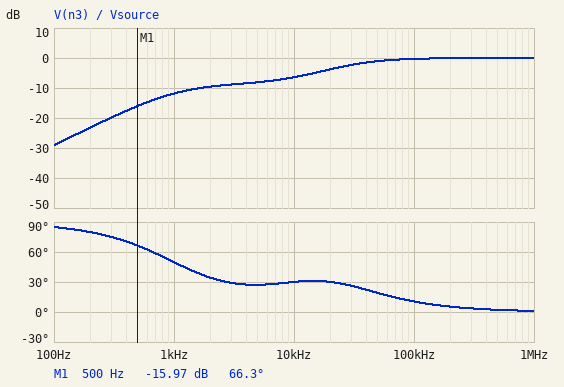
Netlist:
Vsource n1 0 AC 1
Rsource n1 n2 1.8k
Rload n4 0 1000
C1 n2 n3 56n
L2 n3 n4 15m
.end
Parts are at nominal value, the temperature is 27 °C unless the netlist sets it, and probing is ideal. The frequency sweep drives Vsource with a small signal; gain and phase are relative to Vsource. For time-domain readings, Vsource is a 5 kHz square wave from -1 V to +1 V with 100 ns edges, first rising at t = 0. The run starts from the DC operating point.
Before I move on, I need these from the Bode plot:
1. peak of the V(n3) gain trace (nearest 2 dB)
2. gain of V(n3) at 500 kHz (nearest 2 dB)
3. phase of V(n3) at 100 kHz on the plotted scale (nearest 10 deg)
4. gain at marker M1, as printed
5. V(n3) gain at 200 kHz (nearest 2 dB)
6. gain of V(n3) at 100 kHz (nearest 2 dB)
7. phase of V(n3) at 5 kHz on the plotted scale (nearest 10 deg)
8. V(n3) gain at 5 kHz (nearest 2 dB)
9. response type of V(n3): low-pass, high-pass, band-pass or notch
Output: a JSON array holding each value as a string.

["0 dB", "0 dB", "10 deg", "-15.97 dB", "0 dB", "0 dB", "30 deg", "-8 dB", "high-pass"]
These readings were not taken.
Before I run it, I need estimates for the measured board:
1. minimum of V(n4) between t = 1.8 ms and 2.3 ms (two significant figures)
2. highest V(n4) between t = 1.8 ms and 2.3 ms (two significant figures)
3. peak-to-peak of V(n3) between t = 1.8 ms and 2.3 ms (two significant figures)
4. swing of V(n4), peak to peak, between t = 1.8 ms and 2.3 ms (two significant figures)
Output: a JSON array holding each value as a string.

["-420 mV", "420 mV", "3.5 V", "850 mV"]
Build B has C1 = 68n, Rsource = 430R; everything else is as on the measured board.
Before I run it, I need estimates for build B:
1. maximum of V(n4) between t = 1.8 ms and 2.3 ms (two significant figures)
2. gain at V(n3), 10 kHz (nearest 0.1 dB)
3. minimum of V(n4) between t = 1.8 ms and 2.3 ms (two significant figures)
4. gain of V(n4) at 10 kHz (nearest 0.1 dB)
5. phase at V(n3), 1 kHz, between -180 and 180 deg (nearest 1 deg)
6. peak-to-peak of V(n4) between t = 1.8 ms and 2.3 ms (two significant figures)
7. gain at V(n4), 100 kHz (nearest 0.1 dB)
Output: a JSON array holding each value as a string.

["850 mV", "-1.3 dB", "-850 mV", "-4.1 dB", "63 deg", "1.7 V", "-19.6 dB"]
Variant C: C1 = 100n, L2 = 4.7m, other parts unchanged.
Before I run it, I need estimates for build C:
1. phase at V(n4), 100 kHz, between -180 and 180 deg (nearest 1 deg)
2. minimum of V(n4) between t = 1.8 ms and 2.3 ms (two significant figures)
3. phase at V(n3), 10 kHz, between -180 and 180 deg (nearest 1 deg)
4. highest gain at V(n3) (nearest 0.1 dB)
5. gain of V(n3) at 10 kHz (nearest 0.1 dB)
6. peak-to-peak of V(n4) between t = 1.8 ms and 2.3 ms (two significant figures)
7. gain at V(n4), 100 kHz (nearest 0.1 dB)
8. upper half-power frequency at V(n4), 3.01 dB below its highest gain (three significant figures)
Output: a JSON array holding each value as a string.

["-46 deg", "-410 mV", "14 deg", "0 dB", "-8.6 dB", "820 mV", "-12.2 dB", "95.4 kHz"]
